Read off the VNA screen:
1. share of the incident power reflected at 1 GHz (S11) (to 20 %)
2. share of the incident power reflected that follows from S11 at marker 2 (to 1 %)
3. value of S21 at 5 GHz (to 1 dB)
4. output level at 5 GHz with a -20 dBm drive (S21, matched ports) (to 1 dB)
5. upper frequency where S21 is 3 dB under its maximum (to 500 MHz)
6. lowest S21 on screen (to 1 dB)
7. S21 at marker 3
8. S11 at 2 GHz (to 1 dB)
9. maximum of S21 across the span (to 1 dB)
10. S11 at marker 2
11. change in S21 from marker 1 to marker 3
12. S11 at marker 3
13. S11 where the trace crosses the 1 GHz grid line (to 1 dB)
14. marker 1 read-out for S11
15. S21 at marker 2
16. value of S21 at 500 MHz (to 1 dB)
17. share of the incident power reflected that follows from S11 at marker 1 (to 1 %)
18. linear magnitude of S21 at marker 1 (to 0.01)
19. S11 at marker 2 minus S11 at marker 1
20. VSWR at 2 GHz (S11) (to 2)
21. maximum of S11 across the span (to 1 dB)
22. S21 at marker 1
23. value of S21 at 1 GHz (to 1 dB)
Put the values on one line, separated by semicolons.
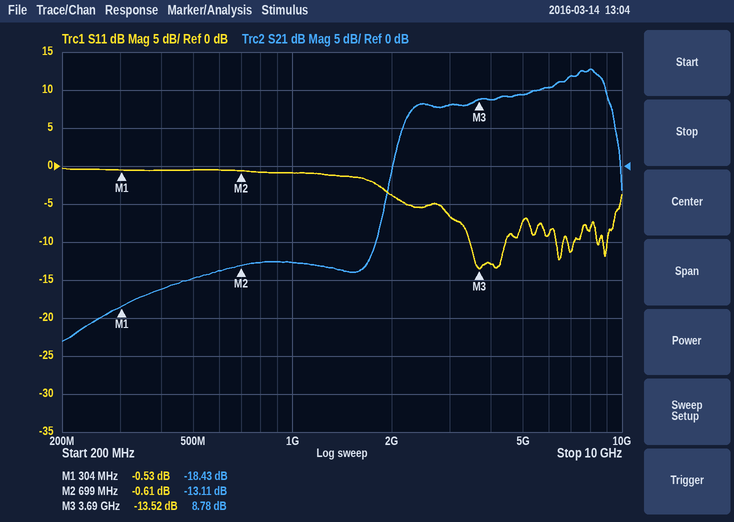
80 %; 87 %; 9 dB; -11 dBm; 9.0 GHz; -23 dB; 8.78 dB; -4 dB; 13 dB; -0.61 dB; 27.21 dB; -13.52 dB; -1 dB; -0.53 dB; -13.11 dB; -15 dB; 89 %; 0.12; -0.08 dB; 4; 0 dB; -18.43 dB; -13 dB
